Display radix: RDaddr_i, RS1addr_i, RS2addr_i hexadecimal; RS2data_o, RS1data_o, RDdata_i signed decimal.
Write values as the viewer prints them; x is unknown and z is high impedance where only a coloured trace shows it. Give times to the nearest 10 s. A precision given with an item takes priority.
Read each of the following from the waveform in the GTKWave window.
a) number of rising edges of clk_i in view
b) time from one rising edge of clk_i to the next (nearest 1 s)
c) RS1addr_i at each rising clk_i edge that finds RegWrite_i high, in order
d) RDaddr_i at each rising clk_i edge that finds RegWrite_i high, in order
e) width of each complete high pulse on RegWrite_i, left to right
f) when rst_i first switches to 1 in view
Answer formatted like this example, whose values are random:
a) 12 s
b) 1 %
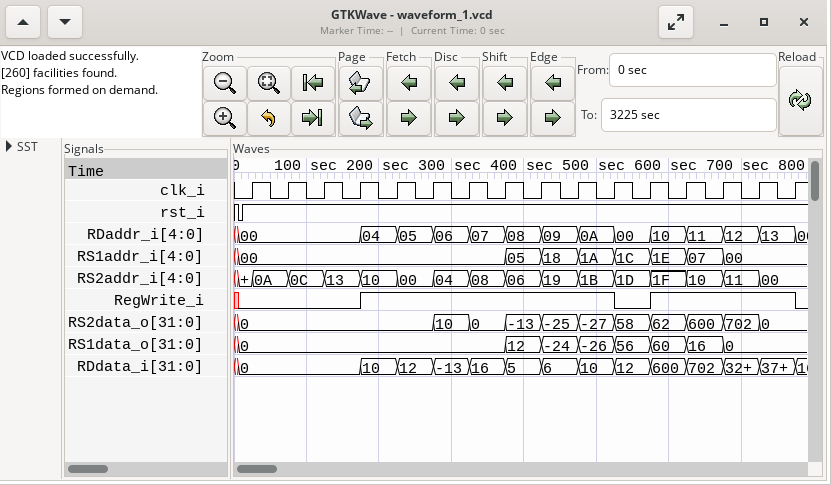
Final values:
a) 16
b) 50 s
c) 00, 00, 00, 00, 05, 18, 1A, 1E, 07, 00, 00
d) 04, 05, 06, 07, 08, 09, 0A, 10, 11, 12, 13
e) 350 s, 200 s
f) 10 s
